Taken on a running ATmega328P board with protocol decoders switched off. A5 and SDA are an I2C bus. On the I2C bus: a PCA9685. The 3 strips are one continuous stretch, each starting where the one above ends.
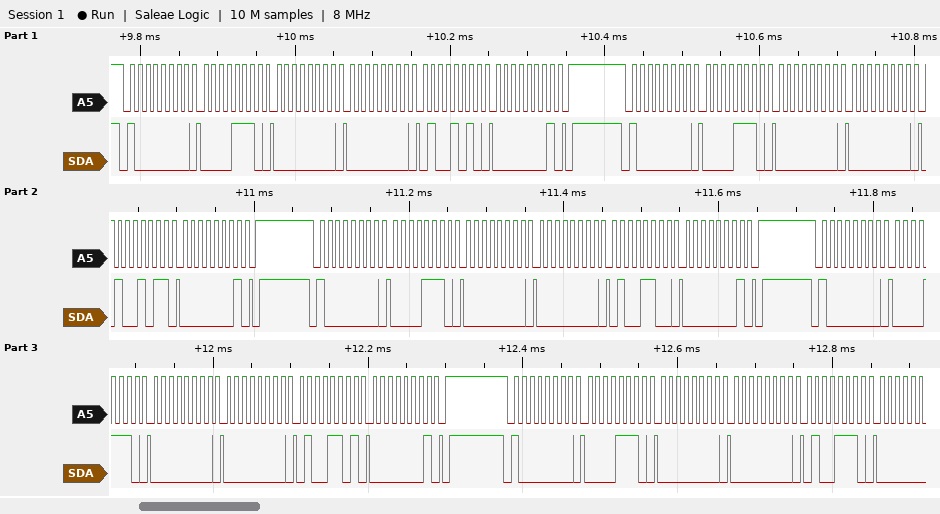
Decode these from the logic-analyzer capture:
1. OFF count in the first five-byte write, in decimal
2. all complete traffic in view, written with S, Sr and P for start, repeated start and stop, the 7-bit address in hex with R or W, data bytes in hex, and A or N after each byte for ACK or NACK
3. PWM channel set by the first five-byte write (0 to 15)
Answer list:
330
S 40W A 0E A 00 A 00 A 4A A 01 A P S 40W A 0E A 00 A 00 A 4B A 01 A P S 40W A 0E A 00 A 00 A 4C A 01 A P S 40W A 0E A 00 A 00 A 4D A 01 A P S 40W A 0E A 00 A 00 A 4E A
2
